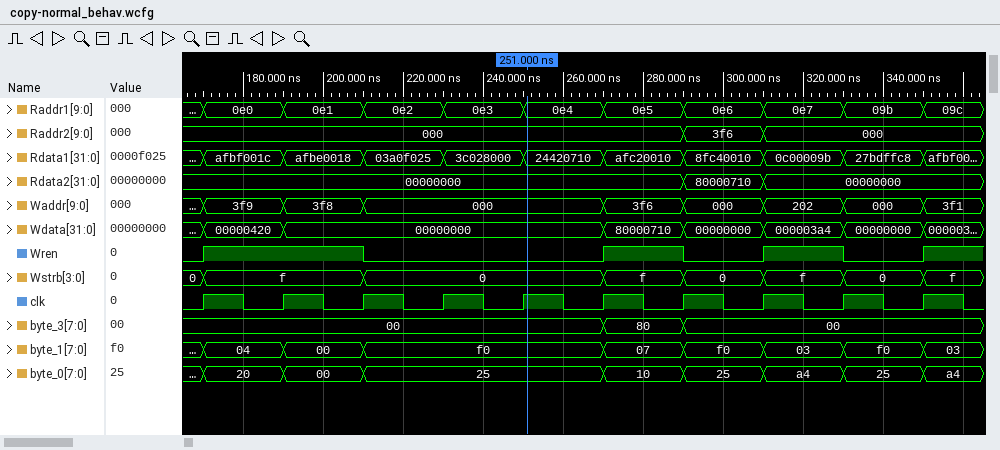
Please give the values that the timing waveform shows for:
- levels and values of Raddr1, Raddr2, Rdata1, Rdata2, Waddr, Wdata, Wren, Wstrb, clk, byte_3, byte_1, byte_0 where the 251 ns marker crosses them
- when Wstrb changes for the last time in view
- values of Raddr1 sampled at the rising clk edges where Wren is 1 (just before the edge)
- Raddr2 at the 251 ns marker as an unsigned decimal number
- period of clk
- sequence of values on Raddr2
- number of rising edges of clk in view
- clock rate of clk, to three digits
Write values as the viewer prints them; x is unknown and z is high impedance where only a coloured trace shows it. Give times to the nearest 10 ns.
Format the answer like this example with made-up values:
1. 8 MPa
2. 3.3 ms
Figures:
1. Raddr1=0e4, Raddr2=000, Rdata1=24420710, Rdata2=00000000, Waddr=000, Wdata=00000000, Wren=0, Wstrb=0, clk=1, byte_3=00, byte_1=f0, byte_0=25
2. 350 ns
3. 0e0, 0e1, 0e5, 0e7
4. 0
5. 20 ns
6. 000, 3f6, 000
7. 10
8. 50.0 MHz
